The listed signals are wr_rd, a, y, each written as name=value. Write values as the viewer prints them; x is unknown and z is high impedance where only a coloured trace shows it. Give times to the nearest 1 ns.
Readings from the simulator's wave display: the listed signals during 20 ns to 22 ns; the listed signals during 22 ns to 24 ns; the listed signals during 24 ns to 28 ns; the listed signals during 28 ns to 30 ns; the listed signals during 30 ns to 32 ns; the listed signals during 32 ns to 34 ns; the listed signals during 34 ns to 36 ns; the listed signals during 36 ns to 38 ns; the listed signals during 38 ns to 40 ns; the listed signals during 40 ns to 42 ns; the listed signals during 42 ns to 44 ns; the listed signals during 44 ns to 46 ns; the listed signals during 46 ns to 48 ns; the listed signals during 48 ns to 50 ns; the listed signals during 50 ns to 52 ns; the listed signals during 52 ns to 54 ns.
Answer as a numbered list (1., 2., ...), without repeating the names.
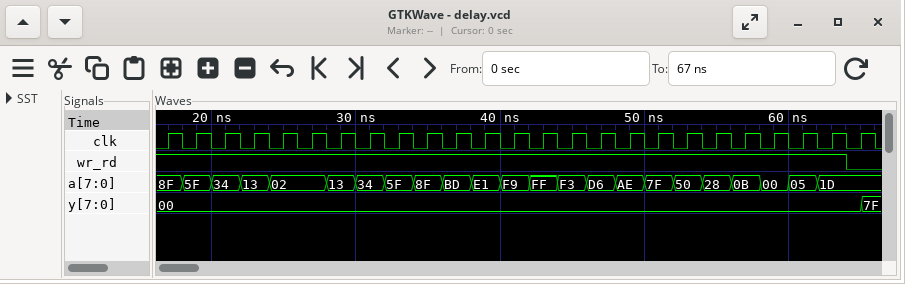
1. wr_rd=1, a=34, y=00
2. wr_rd=1, a=13, y=00
3. wr_rd=1, a=02, y=00
4. wr_rd=1, a=13, y=00
5. wr_rd=1, a=34, y=00
6. wr_rd=1, a=5F, y=00
7. wr_rd=1, a=8F, y=00
8. wr_rd=1, a=BD, y=00
9. wr_rd=1, a=E1, y=00
10. wr_rd=1, a=F9, y=00
11. wr_rd=1, a=FF, y=00
12. wr_rd=1, a=F3, y=00
13. wr_rd=1, a=D6, y=00
14. wr_rd=1, a=AE, y=00
15. wr_rd=1, a=7F, y=00
16. wr_rd=1, a=50, y=00
